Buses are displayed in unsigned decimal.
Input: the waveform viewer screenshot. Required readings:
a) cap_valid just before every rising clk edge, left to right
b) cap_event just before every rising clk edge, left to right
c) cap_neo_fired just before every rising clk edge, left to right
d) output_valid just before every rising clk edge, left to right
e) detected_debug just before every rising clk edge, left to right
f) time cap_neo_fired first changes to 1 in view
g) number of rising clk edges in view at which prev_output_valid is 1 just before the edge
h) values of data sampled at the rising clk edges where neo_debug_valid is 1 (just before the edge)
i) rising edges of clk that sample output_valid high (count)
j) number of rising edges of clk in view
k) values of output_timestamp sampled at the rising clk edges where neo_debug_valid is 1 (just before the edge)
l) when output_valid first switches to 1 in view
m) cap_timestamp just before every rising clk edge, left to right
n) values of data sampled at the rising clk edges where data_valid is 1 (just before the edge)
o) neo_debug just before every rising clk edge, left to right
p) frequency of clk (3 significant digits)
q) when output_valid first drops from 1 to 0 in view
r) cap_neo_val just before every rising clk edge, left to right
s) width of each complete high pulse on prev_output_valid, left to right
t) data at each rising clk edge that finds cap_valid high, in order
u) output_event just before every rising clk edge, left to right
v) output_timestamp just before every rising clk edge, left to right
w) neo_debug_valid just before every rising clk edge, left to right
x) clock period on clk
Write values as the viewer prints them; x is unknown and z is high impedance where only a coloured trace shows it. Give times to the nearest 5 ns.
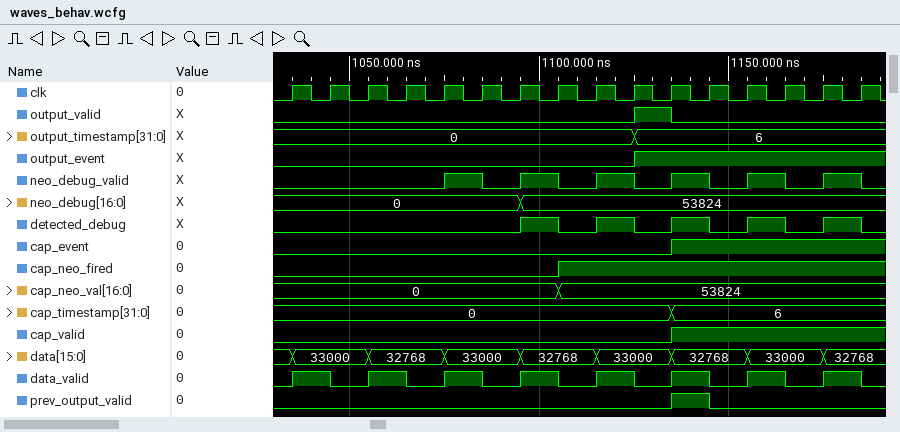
0 0 0 0 0 0 0 0 0 0 0 1 1 1 1 1
0 0 0 0 0 0 0 0 0 0 0 1 1 1 1 1
0 0 0 0 0 0 0 0 1 1 1 1 1 1 1 1
0 0 0 0 0 0 0 0 0 0 1 0 0 0 0 0
0 0 0 0 0 0 0 1 0 1 0 1 0 1 0 1
1105 ns
1
33000, 32768, 33000, 32768, 33000, 32768
1
16
0, 0, 0, 6, 6, 6
1125 ns
0, 0, 0, 0, 0, 0, 0, 0, 0, 0, 0, 6, 6, 6, 6, 6
33000, 32768, 33000, 32768, 33000, 32768, 33000, 32768
0, 0, 0, 0, 0, 0, 0, 53824, 53824, 53824, 53824, 53824, 53824, 53824, 53824, 53824
100 MHz
1135 ns
0, 0, 0, 0, 0, 0, 0, 0, 53824, 53824, 53824, 53824, 53824, 53824, 53824, 53824
10 ns
32768, 32768, 33000, 33000, 32768
0 0 0 0 0 0 0 0 0 0 1 1 1 1 1 1
0, 0, 0, 0, 0, 0, 0, 0, 0, 0, 6, 6, 6, 6, 6, 6
0 0 0 0 0 1 0 1 0 1 0 1 0 1 0 1
10 ns
